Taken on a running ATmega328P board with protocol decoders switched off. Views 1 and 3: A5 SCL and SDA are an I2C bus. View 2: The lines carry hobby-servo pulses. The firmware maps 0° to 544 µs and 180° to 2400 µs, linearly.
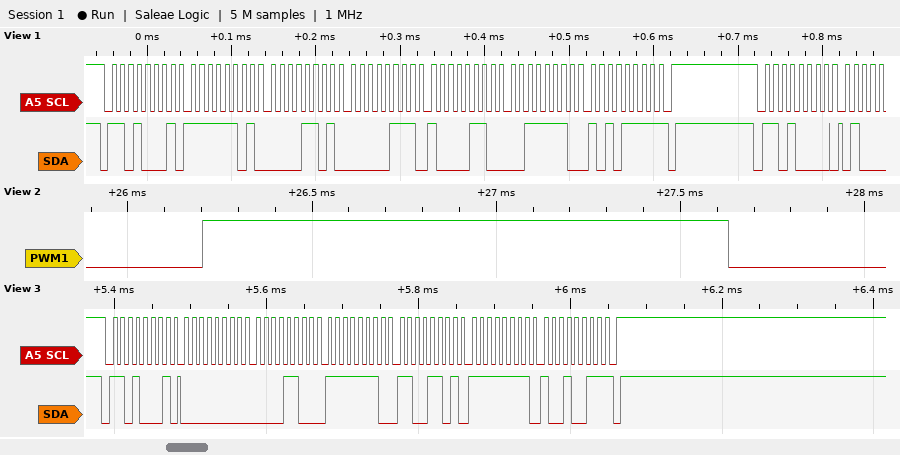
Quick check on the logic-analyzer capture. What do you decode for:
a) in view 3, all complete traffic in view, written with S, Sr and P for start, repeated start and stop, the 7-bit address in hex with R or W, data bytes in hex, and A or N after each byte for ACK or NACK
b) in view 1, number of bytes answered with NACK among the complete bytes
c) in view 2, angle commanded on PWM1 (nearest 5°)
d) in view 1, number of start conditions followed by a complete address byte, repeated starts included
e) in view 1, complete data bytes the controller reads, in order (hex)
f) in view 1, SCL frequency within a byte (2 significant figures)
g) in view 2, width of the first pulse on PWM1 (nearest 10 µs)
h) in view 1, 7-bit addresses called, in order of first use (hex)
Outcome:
S 68R A 00 A 0C A FE A CD A FF A 93 N P
1
85°
2
FD 0D 07 86 3E AF
100 kHz
1430 µs
0x68
